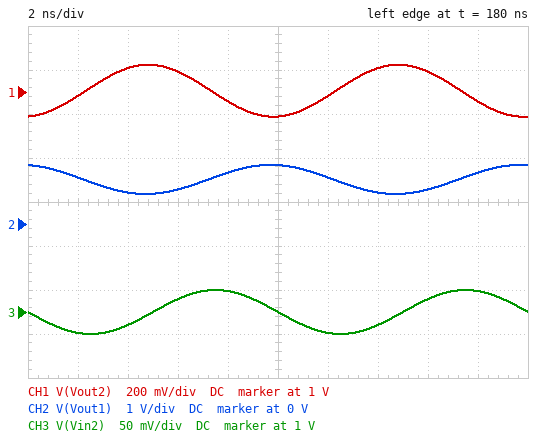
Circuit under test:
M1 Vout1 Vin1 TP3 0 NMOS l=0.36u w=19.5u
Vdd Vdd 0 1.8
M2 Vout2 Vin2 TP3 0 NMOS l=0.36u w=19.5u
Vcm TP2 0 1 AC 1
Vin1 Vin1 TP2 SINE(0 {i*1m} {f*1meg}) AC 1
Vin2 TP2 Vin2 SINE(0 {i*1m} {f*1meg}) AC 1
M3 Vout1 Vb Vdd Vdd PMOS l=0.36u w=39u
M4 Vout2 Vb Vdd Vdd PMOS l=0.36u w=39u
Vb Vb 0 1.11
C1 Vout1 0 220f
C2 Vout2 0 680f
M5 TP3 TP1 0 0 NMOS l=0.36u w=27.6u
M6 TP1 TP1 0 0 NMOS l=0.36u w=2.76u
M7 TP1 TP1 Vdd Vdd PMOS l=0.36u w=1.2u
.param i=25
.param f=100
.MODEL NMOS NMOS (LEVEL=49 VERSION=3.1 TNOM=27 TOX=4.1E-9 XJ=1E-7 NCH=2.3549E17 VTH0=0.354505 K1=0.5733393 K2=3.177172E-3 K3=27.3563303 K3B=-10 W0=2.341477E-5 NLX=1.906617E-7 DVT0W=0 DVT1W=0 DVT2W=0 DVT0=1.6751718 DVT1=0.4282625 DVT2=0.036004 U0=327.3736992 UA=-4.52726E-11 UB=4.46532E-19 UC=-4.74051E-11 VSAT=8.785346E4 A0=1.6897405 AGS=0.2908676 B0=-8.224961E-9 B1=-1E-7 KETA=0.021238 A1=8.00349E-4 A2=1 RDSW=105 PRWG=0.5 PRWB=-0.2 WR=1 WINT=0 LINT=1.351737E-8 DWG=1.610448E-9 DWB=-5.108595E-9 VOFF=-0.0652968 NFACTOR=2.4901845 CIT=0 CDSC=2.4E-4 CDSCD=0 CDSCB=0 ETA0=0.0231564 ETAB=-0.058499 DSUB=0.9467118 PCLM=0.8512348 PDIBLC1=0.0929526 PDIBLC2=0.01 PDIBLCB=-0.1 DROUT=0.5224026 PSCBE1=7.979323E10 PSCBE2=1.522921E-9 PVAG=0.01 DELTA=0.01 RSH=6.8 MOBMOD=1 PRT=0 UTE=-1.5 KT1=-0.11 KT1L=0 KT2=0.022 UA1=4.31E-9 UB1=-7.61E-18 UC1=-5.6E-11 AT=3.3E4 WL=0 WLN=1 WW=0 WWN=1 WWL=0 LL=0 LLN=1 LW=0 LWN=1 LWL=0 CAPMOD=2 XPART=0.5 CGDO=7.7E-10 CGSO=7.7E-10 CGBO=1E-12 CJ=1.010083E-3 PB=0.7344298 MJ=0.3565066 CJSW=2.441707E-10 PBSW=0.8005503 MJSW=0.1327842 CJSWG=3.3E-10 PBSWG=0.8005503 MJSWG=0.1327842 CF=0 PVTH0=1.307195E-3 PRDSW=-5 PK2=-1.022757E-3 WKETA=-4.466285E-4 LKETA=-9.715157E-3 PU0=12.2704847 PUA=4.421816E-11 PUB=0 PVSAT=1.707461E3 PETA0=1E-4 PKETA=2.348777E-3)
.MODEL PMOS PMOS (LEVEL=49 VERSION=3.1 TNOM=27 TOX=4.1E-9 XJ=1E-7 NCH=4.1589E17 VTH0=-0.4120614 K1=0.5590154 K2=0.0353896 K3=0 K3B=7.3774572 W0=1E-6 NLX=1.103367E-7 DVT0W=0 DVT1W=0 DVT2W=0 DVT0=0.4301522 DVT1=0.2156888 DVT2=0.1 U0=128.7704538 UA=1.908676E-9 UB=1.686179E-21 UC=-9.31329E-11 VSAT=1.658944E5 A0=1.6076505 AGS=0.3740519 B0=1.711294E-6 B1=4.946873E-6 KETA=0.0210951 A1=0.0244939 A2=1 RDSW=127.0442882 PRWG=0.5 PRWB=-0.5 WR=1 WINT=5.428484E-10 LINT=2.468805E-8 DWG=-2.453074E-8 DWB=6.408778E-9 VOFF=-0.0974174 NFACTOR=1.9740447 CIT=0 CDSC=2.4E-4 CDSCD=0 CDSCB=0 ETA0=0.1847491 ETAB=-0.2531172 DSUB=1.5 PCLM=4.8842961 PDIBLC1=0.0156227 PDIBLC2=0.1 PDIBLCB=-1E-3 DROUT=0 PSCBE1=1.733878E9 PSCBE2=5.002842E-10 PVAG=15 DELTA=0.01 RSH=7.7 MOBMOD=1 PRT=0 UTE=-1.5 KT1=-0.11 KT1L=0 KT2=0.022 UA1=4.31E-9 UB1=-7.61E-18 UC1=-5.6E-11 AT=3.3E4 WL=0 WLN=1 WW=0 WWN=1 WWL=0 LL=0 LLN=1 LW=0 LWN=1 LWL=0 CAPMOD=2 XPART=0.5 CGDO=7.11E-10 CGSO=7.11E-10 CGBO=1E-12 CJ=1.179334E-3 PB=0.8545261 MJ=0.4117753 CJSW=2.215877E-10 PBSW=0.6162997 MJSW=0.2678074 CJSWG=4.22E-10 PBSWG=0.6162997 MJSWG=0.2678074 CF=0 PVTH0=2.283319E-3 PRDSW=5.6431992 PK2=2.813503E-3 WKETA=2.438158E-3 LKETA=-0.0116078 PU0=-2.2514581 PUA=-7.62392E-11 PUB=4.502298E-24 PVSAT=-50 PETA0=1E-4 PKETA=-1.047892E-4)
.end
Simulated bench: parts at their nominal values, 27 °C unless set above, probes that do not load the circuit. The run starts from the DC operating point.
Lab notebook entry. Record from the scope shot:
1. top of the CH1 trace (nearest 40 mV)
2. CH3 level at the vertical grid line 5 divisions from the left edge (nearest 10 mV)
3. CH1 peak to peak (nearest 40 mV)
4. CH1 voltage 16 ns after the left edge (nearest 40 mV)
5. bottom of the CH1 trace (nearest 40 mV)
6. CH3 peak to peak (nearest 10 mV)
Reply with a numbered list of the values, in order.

1. 1.12 V
2. 1.00 V
3. 240 mV
4. 1.08 V
5. 880 mV
6. 50 mV
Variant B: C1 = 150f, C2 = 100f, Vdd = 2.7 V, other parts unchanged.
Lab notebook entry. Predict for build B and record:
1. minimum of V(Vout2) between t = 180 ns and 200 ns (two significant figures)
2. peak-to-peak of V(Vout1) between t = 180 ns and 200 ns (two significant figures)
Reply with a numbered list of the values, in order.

1. 2.6 V
2. 29 mV
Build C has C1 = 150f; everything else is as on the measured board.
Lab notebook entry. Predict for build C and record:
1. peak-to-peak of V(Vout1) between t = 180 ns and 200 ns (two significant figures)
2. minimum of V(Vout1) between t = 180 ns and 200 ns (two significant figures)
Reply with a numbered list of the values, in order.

1. 890 mV
2. 570 mV
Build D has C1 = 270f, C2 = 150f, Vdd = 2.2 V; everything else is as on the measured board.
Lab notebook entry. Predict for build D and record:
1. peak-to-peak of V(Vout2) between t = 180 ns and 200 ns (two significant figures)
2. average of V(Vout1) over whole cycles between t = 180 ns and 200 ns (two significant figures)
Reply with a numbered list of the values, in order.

1. 42 mV
2. 2.1 V
